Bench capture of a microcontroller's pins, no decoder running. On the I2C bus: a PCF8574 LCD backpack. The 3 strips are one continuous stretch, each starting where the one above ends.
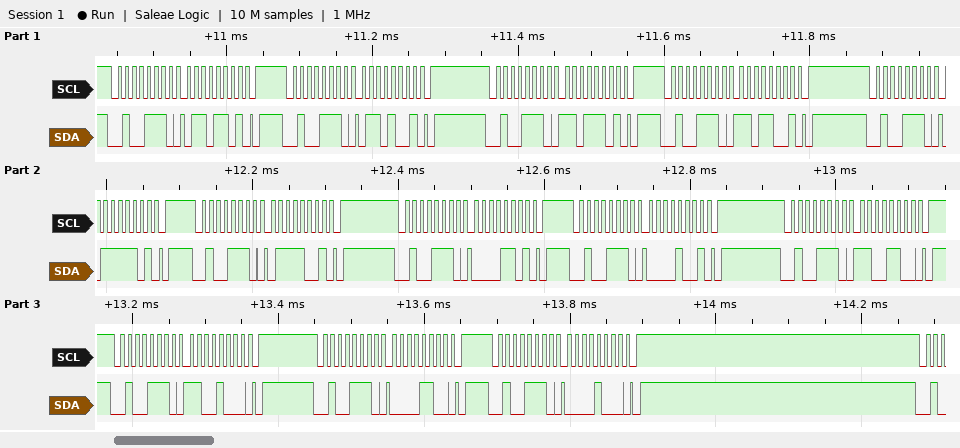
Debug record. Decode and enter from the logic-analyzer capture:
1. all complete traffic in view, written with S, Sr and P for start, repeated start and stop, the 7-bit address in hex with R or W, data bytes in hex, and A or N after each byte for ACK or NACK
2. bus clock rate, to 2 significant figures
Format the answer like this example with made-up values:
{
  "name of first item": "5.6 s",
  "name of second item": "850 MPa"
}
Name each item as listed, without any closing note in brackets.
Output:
{
  "all complete traffic in view, written with S, Sr and P for start, repeated start and stop, the 7-bit address in hex with R or W, data bytes in hex, and A or N after each byte for ACK or NACK": "S 27W A 6D A P S 27W A 69 A P S 27W A DD A P S 27W A D9 A P S 27W A 7D A P S 27W A 79 A P S 27W A 0D A P S 27W A 09 A P S 27W A CC A P S 27W A C8 A P S 27W A 0C A P S 27W A 08 A P",
  "bus clock rate, to 2 significant figures": "100 kHz"
}
